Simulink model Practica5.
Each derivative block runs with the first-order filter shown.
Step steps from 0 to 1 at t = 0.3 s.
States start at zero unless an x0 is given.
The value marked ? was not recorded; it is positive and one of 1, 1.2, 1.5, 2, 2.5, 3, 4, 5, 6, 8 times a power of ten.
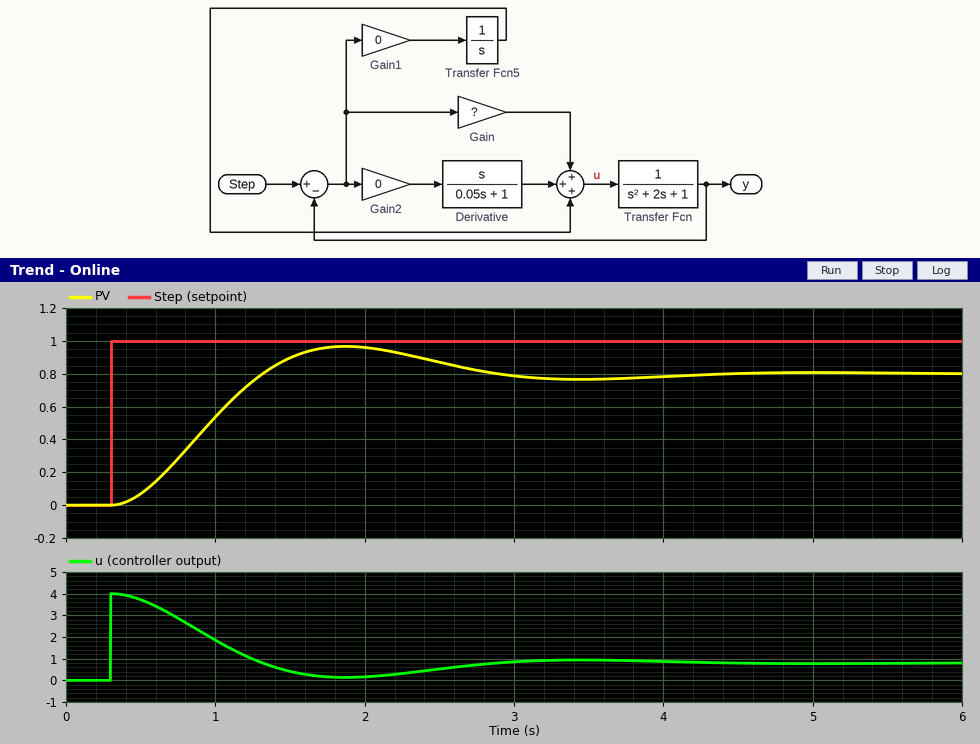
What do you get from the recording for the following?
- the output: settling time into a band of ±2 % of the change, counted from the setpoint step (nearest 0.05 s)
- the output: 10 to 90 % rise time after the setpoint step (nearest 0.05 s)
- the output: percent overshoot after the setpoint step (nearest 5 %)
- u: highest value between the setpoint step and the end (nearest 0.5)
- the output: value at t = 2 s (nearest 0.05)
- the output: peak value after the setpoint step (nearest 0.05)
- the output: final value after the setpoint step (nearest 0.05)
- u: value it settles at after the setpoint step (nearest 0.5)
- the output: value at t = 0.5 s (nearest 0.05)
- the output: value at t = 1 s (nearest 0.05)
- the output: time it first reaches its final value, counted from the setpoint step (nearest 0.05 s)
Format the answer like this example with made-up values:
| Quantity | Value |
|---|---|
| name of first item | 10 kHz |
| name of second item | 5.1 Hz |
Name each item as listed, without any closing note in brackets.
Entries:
| Quantity | Value |
|---|---|
| the output: settling time into a band of ±2 % of the change, counted from the setpoint step | 3.75 s |
| the output: 10 to 90 % rise time after the setpoint step | 0.70 s |
| the output: percent overshoot after the setpoint step | 20 % |
| u: highest value between the setpoint step and the end | 4.0 |
| the output: value at t = 2 s | 0.95 |
| the output: peak value after the setpoint step | 0.95 |
| the output: final value after the setpoint step | 0.80 |
| u: value it settles at after the setpoint step | 1.0 |
| the output: value at t = 0.5 s | 0.05 |
| the output: value at t = 1 s | 0.55 |
| the output: time it first reaches its final value, counted from the setpoint step | 1.00 s |
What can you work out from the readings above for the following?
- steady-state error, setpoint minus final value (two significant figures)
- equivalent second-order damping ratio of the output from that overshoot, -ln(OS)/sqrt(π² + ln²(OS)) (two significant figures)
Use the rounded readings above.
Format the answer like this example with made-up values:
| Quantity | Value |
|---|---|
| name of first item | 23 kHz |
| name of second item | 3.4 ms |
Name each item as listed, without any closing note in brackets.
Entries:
| Quantity | Value |
|---|---|
| steady-state error, setpoint minus final value | 0.20 |
| equivalent second-order damping ratio of the output from that overshoot, -ln(OS)/sqrt(π² + ln²(OS)) | 0.46 |
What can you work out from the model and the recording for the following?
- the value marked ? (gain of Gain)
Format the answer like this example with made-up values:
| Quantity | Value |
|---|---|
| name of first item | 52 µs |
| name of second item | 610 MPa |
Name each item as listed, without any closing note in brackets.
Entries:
| Quantity | Value |
|---|---|
| the value marked ? | 4 |
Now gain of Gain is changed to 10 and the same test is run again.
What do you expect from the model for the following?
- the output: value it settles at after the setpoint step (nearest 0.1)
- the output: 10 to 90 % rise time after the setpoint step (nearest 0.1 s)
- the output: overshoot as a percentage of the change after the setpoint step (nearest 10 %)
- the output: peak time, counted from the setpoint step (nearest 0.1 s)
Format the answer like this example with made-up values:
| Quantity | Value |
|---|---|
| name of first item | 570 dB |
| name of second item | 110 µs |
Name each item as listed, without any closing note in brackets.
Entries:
| Quantity | Value |
|---|---|
| the output: value it settles at after the setpoint step | 0.9 |
| the output: 10 to 90 % rise time after the setpoint step | 0.4 s |
| the output: overshoot as a percentage of the change after the setpoint step | 40 % |
| the output: peak time, counted from the setpoint step | 1.0 s |
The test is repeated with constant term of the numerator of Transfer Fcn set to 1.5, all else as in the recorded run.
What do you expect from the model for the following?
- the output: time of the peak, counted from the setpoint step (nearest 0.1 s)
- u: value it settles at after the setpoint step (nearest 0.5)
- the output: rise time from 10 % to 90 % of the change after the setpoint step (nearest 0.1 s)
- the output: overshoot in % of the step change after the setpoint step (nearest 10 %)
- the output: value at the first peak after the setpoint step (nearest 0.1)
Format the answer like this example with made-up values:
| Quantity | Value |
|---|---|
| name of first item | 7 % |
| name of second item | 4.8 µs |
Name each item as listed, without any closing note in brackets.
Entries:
| Quantity | Value |
|---|---|
| the output: time of the peak, counted from the setpoint step | 1.3 s |
| u: value it settles at after the setpoint step | 0.5 |
| the output: rise time from 10 % to 90 % of the change after the setpoint step | 0.5 s |
| the output: overshoot in % of the step change after the setpoint step | 30 % |
| the output: value at the first peak after the setpoint step | 1.1 |
